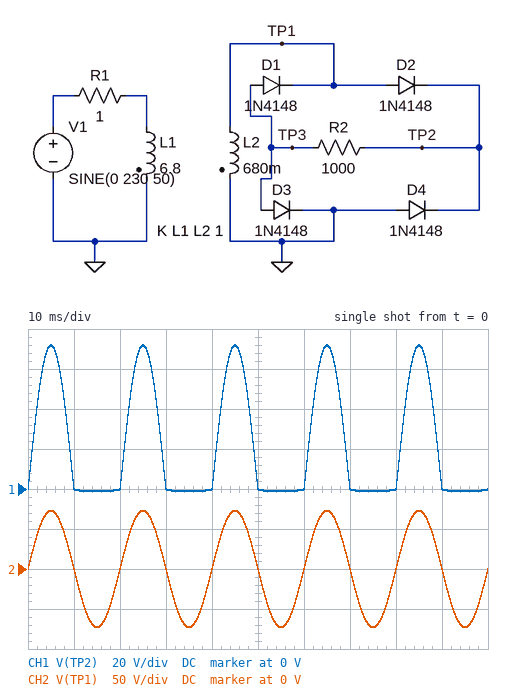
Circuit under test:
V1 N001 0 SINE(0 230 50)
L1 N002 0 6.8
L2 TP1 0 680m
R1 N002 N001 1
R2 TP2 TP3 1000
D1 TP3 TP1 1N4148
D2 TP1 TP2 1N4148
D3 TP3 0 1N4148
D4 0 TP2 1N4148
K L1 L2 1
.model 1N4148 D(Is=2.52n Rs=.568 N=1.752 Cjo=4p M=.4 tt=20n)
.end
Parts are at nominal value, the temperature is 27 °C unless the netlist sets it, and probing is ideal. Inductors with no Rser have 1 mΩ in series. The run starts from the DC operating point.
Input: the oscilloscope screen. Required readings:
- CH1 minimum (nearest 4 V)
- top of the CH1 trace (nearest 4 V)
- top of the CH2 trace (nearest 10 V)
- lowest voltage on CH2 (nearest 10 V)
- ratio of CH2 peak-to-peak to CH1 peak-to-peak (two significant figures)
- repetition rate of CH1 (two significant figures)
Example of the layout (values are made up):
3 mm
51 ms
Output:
0 V
72 V
70 V
-70 V
2.0
50 Hz
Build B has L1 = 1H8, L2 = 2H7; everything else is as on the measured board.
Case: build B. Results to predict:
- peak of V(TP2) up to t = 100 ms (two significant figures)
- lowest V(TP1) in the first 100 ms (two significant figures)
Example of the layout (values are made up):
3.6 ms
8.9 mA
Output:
280 V
-280 V
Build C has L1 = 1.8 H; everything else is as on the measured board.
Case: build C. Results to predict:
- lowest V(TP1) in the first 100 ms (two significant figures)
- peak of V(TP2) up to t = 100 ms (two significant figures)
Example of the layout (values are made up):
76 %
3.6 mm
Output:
-140 V
140 V
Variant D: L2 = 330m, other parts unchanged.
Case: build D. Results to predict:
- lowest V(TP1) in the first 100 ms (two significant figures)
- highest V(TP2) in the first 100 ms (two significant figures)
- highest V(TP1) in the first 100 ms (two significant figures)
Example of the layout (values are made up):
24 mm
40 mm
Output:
-51 V
50 V
51 V
